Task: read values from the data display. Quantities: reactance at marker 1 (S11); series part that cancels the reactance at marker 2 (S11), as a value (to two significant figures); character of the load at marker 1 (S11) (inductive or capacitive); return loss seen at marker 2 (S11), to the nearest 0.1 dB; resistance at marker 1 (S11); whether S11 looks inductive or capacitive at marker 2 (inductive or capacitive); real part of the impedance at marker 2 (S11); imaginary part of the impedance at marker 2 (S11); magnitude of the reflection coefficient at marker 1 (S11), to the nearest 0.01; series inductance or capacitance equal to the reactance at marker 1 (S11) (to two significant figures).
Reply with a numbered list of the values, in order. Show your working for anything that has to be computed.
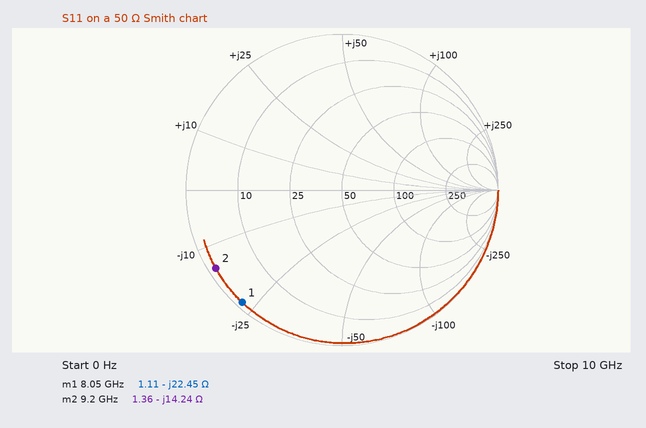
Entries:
1. -22.45 Ω
2. L = 14.24 Ω/(2π × 9.2 GHz) ≈ 246 pH, so 250 pH to two significant figures
3. capacitive
4. 0.4 dB
5. 1.11 Ω
6. capacitive
7. 1.36 Ω
8. -14.24 Ω
9. 0.96
10. C = 1/(2π × 8.05 GHz × 22.45 Ω) ≈ 881 fF, so 880 fF to two significant figures
